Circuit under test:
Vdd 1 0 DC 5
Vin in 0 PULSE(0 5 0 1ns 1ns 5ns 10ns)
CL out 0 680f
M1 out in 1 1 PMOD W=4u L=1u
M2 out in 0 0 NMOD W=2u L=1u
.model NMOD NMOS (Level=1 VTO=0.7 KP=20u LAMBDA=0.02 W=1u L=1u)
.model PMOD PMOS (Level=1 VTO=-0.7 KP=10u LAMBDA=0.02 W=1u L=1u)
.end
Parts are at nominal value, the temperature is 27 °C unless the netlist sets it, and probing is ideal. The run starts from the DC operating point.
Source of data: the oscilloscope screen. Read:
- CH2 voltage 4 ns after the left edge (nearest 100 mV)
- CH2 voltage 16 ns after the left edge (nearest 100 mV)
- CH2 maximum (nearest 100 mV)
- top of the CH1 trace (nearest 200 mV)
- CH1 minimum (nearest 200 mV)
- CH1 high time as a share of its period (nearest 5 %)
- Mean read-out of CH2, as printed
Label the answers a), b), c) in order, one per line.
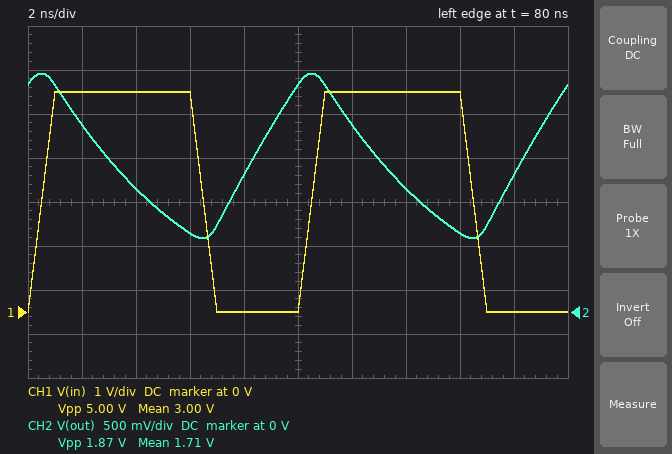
a) 1.4 V
b) 900 mV
c) 2.7 V
d) 5.0 V
e) 0 V
f) 60 %
g) 1.71 V
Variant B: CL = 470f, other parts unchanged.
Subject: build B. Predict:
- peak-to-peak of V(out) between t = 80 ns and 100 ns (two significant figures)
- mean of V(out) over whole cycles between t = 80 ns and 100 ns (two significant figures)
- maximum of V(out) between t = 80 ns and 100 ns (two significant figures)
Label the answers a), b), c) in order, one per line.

a) 2.6 V
b) 1.8 V
c) 3.2 V
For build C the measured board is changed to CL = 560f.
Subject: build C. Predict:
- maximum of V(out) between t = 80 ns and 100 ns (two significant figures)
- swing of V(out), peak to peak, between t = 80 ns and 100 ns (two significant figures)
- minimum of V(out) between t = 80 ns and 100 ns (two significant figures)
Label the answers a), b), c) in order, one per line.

a) 2.9 V
b) 2.2 V
c) 710 mV
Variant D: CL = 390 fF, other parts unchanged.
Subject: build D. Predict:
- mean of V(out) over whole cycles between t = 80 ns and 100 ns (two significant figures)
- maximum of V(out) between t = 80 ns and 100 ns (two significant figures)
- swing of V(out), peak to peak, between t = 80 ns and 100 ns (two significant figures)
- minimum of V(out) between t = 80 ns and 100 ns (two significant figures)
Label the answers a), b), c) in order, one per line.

a) 1.8 V
b) 3.5 V
c) 3.0 V
d) 450 mV
